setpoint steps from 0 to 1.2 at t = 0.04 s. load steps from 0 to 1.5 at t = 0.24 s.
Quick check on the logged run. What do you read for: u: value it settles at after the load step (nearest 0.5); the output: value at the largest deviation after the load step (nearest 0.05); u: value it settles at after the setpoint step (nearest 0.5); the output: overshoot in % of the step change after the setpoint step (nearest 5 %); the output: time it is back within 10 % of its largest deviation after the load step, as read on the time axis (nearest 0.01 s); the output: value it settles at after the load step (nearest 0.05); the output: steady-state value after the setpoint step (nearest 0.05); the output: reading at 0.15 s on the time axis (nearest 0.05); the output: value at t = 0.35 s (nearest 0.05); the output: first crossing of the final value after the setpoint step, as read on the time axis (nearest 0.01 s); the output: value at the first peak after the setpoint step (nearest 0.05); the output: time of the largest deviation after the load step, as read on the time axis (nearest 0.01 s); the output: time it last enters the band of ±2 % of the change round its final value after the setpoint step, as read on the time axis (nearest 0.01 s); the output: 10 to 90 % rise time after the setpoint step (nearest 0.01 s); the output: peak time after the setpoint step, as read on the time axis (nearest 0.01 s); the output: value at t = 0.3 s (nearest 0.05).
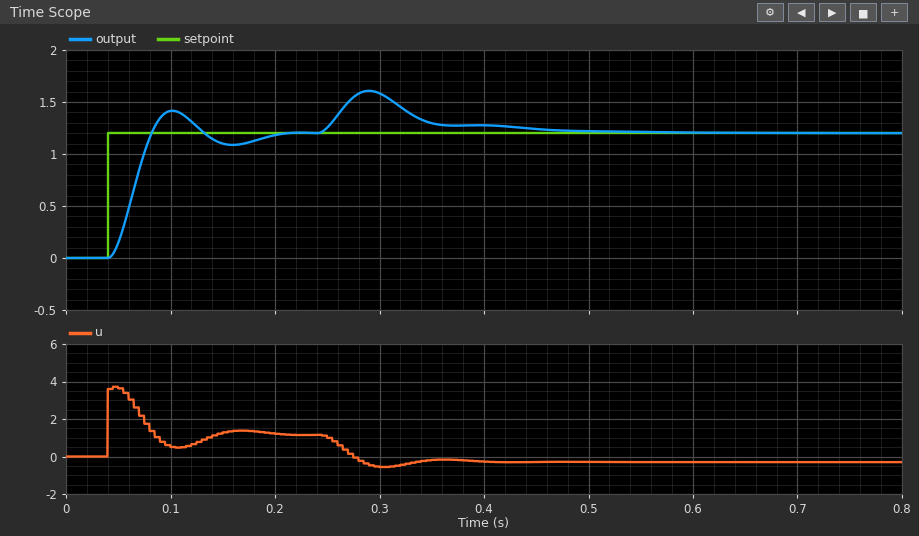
-0.5
1.60
1.0
20 %
0.45 s
1.20
1.20
1.10
1.30
0.08 s
1.40
0.29 s
0.20 s
0.03 s
0.10 s
1.60
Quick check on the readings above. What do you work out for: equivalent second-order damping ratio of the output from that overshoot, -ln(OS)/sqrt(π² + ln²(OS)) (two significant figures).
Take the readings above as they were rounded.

0.46
